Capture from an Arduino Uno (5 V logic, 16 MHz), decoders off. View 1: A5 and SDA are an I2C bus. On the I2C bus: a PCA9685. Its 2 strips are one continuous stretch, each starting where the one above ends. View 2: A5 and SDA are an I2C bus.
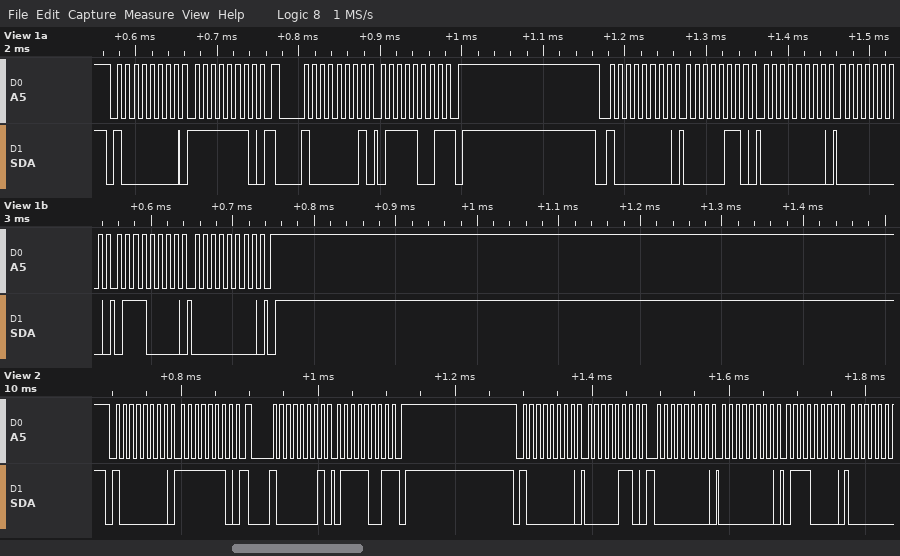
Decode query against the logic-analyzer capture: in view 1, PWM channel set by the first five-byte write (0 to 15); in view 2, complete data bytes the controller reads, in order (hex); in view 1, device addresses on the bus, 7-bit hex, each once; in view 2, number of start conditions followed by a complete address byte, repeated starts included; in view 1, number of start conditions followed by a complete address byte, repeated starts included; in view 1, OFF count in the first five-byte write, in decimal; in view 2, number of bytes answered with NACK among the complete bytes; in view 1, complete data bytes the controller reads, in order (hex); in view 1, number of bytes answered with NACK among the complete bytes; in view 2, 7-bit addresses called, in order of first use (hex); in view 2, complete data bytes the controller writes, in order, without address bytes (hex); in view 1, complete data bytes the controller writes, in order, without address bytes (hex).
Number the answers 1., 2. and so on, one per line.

1. 0
2. 79
3. 0x40
4. 3
5. 3
6. 112
7. 1
8. 79
9. 1
10. 0x40
11. FE 06 00 00 70
12. FE 06 00 00 70 00
